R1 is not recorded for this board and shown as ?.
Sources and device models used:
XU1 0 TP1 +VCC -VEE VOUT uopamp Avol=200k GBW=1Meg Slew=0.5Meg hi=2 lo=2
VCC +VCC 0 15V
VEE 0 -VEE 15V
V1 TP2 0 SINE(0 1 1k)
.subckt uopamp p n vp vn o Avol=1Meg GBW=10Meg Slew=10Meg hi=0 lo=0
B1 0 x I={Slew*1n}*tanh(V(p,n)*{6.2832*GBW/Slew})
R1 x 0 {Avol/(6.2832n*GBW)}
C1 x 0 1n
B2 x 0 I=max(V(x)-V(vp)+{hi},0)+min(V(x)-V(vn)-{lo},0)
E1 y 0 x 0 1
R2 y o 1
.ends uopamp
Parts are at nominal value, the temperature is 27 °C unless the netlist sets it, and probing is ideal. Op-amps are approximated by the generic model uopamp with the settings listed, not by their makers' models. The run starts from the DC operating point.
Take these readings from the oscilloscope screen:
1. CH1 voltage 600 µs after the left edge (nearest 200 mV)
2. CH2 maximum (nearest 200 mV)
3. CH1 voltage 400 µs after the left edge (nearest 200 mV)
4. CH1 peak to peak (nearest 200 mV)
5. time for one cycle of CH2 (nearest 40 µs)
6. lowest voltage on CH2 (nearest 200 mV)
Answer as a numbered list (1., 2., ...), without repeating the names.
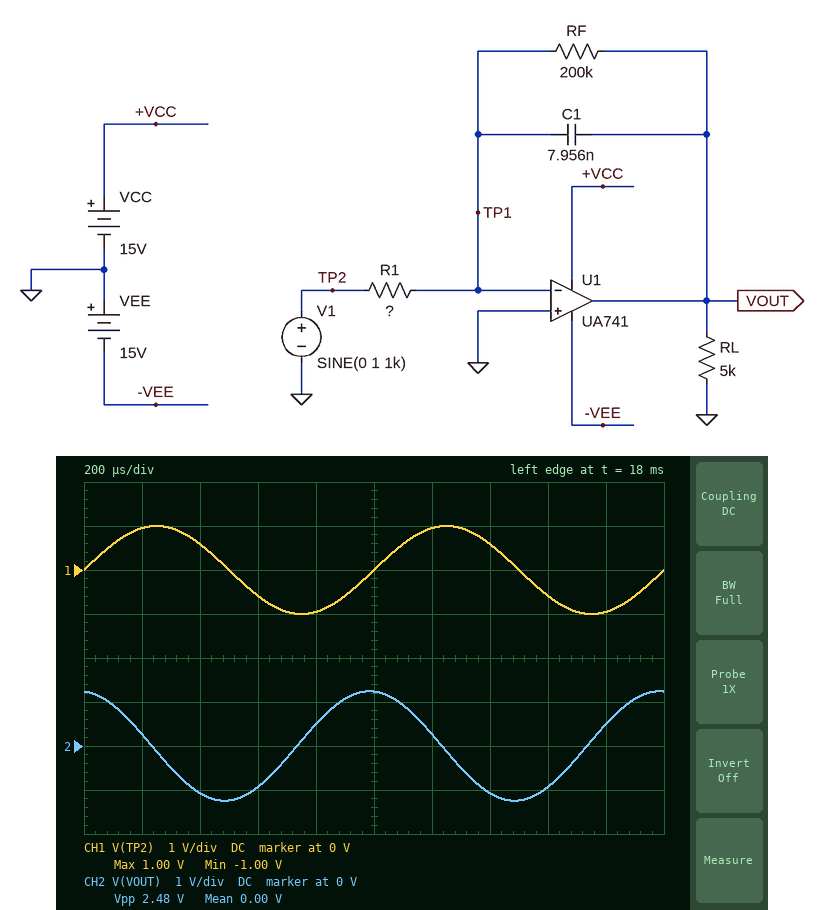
1. -600 mV
2. 1.2 V
3. 600 mV
4. 2.0 V
5. 1.00 ms
6. -1.2 V
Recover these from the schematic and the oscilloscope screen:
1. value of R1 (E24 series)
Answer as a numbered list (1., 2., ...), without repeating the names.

1. 16 kΩ
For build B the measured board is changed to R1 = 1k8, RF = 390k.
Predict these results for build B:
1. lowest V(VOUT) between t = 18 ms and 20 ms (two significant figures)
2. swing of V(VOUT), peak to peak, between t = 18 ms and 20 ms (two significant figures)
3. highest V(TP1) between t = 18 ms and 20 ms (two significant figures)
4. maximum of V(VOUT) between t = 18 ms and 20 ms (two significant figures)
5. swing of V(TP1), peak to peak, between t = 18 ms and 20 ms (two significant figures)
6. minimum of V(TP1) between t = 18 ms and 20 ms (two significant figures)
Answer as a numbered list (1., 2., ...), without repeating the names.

1. -11 V
2. 22 V
3. 11 mV
4. 11 V
5. 22 mV
6. -11 mV
